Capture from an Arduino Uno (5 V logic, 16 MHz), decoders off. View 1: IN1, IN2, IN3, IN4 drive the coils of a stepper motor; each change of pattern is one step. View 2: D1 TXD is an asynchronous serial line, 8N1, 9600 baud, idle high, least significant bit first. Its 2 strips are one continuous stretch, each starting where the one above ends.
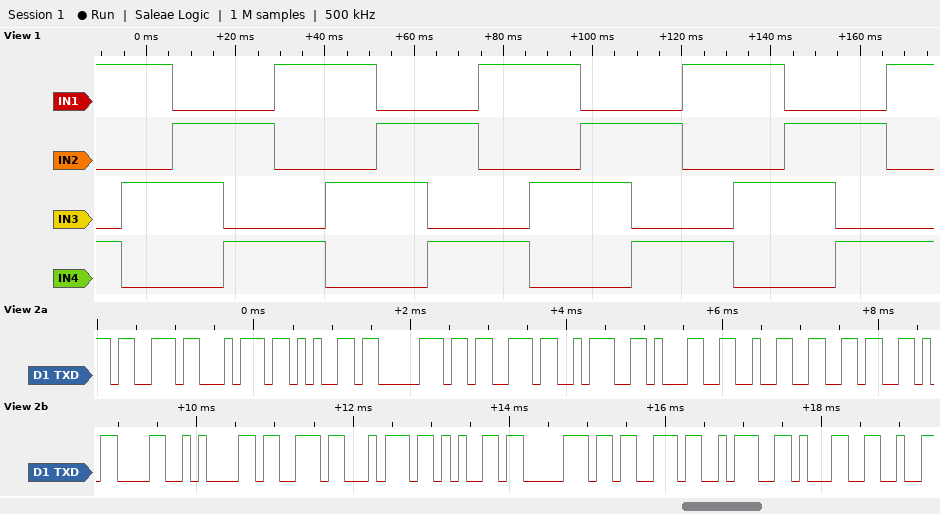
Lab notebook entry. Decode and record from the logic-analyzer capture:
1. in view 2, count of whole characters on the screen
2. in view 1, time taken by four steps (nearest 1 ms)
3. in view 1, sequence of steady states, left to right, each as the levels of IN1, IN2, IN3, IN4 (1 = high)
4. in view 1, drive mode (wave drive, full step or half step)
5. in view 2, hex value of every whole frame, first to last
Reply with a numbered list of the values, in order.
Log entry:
1. 18
2. 46 ms
3. 1001 1010 0110 0101 1001 1010 0110 0101 1001 1010 0110 0101 1001 1010 0110 0101 1001
4. full step
5. 73 74 65 70 73 3A 31 32 36 0D 0A 73 74 65 70 73 3A 31
